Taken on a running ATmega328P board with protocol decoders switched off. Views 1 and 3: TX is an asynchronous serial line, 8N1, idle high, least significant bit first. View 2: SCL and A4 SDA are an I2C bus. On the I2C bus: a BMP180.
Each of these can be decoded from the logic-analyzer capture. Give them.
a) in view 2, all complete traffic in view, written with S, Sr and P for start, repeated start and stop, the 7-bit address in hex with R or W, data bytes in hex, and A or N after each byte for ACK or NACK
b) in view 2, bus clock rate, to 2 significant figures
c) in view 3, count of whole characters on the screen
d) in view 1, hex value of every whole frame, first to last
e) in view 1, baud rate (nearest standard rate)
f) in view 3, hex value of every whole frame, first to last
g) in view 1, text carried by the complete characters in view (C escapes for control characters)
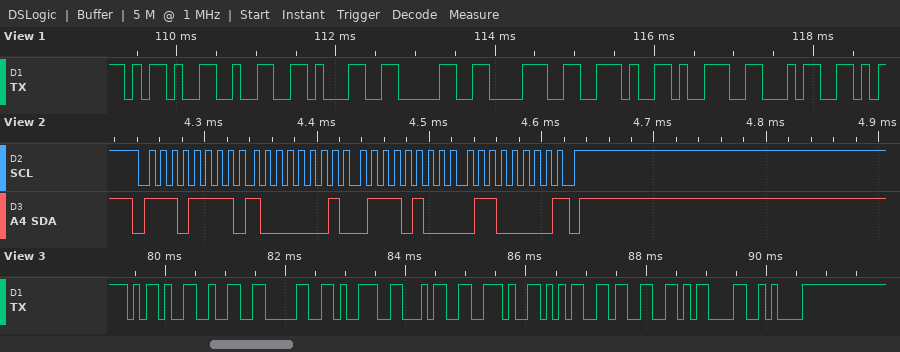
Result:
S 77R A 81 A 74 A 60 N P
100 kHz
10
2D 32 31 30 38 2E 39 34
9600 baud
0x2D 0x32 0x30 0x39 0x34 0x2E 0x35 0x33 0x0D 0x0A
"-2108.94"
